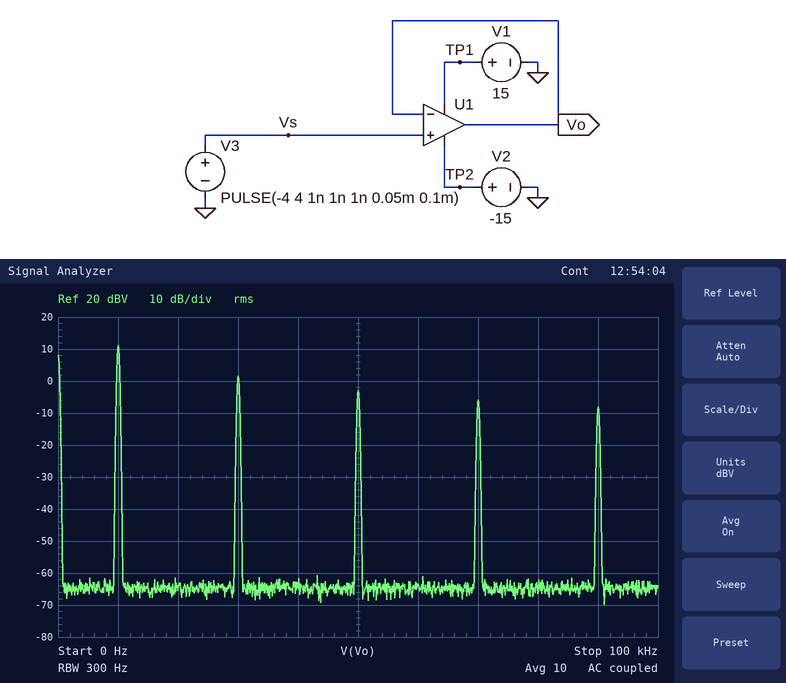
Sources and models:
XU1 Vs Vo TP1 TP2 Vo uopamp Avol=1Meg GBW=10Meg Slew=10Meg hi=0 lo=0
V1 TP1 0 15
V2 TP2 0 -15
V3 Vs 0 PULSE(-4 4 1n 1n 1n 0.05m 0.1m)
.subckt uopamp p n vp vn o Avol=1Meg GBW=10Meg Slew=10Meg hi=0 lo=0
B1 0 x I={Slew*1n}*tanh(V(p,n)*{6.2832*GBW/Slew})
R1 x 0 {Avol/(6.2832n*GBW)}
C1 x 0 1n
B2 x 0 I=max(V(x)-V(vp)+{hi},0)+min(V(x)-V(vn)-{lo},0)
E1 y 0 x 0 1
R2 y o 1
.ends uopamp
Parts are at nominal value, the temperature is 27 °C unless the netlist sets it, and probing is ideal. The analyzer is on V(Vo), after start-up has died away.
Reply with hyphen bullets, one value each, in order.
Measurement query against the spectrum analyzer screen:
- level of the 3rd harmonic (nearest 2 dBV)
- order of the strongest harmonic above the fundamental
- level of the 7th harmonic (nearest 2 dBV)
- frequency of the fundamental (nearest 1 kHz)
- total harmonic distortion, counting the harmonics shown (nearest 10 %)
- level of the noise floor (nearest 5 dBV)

- 2 dBV
- 3
- -6 dBV
- 10 kHz
- 40 %
- -65 dBV
